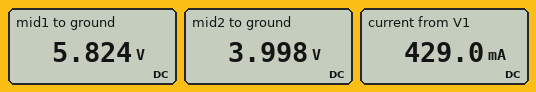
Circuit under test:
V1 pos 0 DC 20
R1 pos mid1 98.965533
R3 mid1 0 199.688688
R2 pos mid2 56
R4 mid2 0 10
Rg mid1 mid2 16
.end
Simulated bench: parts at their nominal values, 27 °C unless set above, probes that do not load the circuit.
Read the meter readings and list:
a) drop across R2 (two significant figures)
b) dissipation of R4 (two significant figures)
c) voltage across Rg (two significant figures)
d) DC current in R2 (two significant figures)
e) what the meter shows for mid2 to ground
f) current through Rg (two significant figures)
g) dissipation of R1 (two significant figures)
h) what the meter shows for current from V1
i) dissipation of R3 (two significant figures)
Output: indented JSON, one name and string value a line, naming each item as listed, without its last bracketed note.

{
  "drop across R2": "16 V",
  "dissipation of R4": "1.6 W",
  "voltage across Rg": "1.8 V",
  "DC current in R2": "290 mA",
  "what the meter shows for mid2 to ground": "3.998 V",
  "current through Rg": "110 mA",
  "dissipation of R1": "2.0 W",
  "what the meter shows for current from V1": "429.0 mA",
  "dissipation of R3": "170 mW"
}
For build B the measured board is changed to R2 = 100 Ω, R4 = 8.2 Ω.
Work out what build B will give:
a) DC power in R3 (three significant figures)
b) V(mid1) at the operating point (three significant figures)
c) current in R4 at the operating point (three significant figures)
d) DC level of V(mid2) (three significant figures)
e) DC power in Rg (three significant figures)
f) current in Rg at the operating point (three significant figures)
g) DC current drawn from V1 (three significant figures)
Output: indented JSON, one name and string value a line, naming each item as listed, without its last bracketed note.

{
  "DC power in R3": "107 mW",
  "V(mid1) at the operating point": "4.63 V",
  "current in R4 at the operating point": "307 mA",
  "DC level of V(mid2)": "2.52 V",
  "DC power in Rg": "279 mW",
  "current in Rg at the operating point": "132 mA",
  "DC current drawn from V1": "330 mA"
}
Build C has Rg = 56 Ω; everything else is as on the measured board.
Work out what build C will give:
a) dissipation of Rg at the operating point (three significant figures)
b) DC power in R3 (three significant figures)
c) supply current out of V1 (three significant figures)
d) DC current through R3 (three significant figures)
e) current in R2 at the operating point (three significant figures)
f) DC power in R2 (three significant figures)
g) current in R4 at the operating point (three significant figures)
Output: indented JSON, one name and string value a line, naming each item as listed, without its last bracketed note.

{
  "dissipation of Rg at the operating point": "351 mW",
  "DC power in R3": "331 mW",
  "supply current out of V1": "411 mA",
  "DC current through R3": "40.7 mA",
  "current in R2 at the operating point": "291 mA",
  "DC power in R2": "4.74 W",
  "current in R4 at the operating point": "370 mA"
}
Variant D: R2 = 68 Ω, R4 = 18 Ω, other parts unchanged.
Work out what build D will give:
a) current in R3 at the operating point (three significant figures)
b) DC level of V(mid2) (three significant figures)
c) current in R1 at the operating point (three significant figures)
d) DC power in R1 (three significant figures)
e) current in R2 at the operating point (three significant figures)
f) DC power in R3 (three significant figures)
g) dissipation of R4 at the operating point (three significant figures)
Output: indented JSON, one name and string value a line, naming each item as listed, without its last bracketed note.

{
  "current in R3 at the operating point": "35.4 mA",
  "DC level of V(mid2)": "5.54 V",
  "current in R1 at the operating point": "131 mA",
  "DC power in R1": "1.69 W",
  "current in R2 at the operating point": "213 mA",
  "DC power in R3": "250 mW",
  "dissipation of R4 at the operating point": "1.71 W"
}
